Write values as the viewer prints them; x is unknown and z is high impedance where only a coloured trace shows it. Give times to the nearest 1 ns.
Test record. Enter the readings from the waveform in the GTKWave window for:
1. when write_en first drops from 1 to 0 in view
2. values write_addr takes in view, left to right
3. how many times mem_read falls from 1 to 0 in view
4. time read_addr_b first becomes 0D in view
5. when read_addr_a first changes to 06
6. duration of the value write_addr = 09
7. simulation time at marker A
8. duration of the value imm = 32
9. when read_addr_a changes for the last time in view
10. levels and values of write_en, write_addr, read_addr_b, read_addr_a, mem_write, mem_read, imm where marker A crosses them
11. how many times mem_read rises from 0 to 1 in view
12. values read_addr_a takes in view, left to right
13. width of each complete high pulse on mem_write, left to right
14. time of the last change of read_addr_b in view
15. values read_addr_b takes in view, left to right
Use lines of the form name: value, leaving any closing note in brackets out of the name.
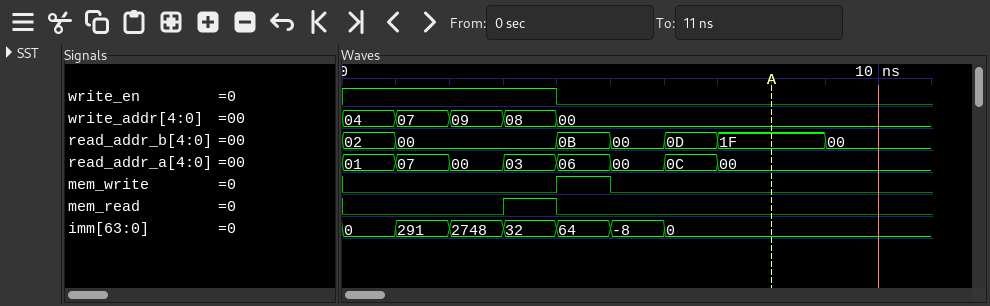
when write_en first drops from 1 to 0 in view: 4 ns
values write_addr takes in view, left to right: 04, 07, 09, 08, 00
how many times mem_read falls from 1 to 0 in view: 1
time read_addr_b first becomes 0D in view: 6 ns
when read_addr_a first changes to 06: 4 ns
duration of the value write_addr = 09: 1 ns
simulation time at marker A: 8 ns
duration of the value imm = 32: 1 ns
when read_addr_a changes for the last time in view: 7 ns
levels and values of write_en, write_addr, read_addr_b, read_addr_a, mem_write, mem_read, imm where marker A crosses them: write_en=0, write_addr=00, read_addr_b=1F, read_addr_a=00, mem_write=0, mem_read=0, imm=0
how many times mem_read rises from 0 to 1 in view: 1
values read_addr_a takes in view, left to right: 01, 07, 00, 03, 06, 00, 0C, 00
width of each complete high pulse on mem_write, left to right: 1 ns
time of the last change of read_addr_b in view: 9 ns
values read_addr_b takes in view, left to right: 02, 00, 0B, 00, 0D, 1F, 00
